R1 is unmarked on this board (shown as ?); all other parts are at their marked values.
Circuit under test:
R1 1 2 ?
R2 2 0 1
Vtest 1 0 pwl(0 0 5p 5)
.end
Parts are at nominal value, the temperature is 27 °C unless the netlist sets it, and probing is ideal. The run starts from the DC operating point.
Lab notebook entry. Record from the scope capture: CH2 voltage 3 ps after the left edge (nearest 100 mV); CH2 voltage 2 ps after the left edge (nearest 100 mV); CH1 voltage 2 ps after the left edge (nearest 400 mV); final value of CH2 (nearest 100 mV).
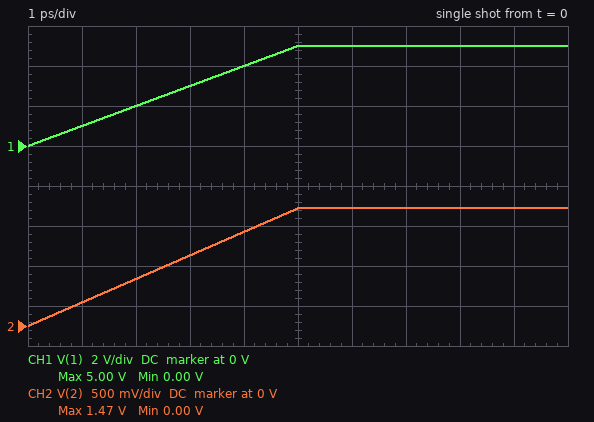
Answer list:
900 mV
600 mV
2.0 V
1.5 V
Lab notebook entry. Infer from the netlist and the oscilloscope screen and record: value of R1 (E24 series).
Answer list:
2.4 Ω
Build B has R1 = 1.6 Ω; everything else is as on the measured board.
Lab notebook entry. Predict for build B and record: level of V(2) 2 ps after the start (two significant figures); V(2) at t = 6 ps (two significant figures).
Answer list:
770 mV
1.9 V
